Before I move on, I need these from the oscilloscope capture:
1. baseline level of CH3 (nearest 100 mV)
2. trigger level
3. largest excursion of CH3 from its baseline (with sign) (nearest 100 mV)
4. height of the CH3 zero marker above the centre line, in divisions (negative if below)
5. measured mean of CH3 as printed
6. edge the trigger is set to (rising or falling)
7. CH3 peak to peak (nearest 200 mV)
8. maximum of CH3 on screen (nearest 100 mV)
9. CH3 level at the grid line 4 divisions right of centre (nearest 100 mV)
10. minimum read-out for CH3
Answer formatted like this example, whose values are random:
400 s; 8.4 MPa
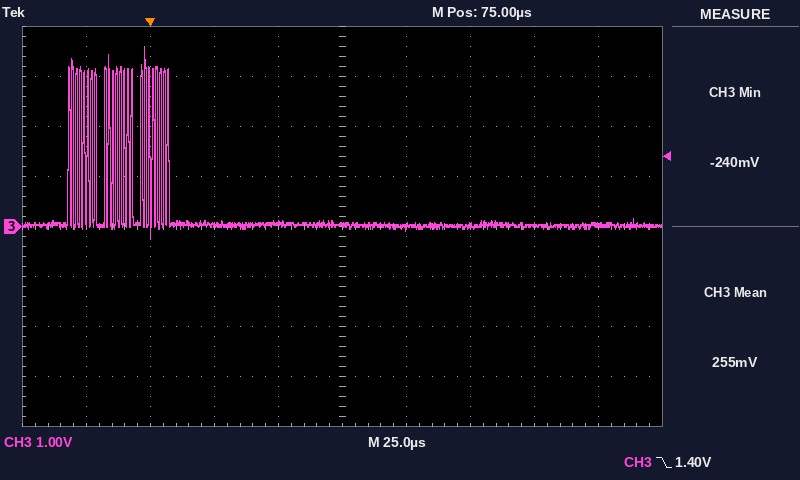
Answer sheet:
0.0 V; 1.40 V; +3.6 V; 0.0 div; 255 mV; falling; 3.8 V; 3.6 V; 0.0 V; -240 mV
